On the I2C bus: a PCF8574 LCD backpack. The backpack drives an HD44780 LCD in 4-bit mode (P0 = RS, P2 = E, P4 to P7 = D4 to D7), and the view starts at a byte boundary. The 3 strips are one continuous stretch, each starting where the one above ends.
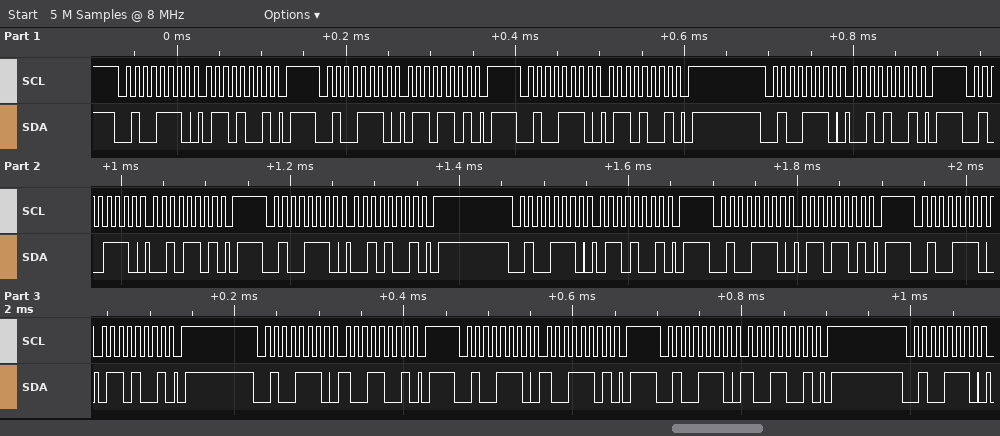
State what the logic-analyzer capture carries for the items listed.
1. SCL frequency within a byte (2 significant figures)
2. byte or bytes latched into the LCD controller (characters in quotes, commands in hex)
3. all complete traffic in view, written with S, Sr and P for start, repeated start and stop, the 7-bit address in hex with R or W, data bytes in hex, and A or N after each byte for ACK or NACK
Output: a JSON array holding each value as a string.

["100 kHz", "'b' 'i'", "S 27W A 69 A P S 27W A 6D A P S 27W A 69 A P S 27W A 29 A P S 27W A 2D A P S 27W A 29 A P S 27W A 69 A P S 27W A 6D A P S 27W A 69 A P S 27W A 99 A P S 27W A 9D A P S 27W A 99 A P S 27W A"]
